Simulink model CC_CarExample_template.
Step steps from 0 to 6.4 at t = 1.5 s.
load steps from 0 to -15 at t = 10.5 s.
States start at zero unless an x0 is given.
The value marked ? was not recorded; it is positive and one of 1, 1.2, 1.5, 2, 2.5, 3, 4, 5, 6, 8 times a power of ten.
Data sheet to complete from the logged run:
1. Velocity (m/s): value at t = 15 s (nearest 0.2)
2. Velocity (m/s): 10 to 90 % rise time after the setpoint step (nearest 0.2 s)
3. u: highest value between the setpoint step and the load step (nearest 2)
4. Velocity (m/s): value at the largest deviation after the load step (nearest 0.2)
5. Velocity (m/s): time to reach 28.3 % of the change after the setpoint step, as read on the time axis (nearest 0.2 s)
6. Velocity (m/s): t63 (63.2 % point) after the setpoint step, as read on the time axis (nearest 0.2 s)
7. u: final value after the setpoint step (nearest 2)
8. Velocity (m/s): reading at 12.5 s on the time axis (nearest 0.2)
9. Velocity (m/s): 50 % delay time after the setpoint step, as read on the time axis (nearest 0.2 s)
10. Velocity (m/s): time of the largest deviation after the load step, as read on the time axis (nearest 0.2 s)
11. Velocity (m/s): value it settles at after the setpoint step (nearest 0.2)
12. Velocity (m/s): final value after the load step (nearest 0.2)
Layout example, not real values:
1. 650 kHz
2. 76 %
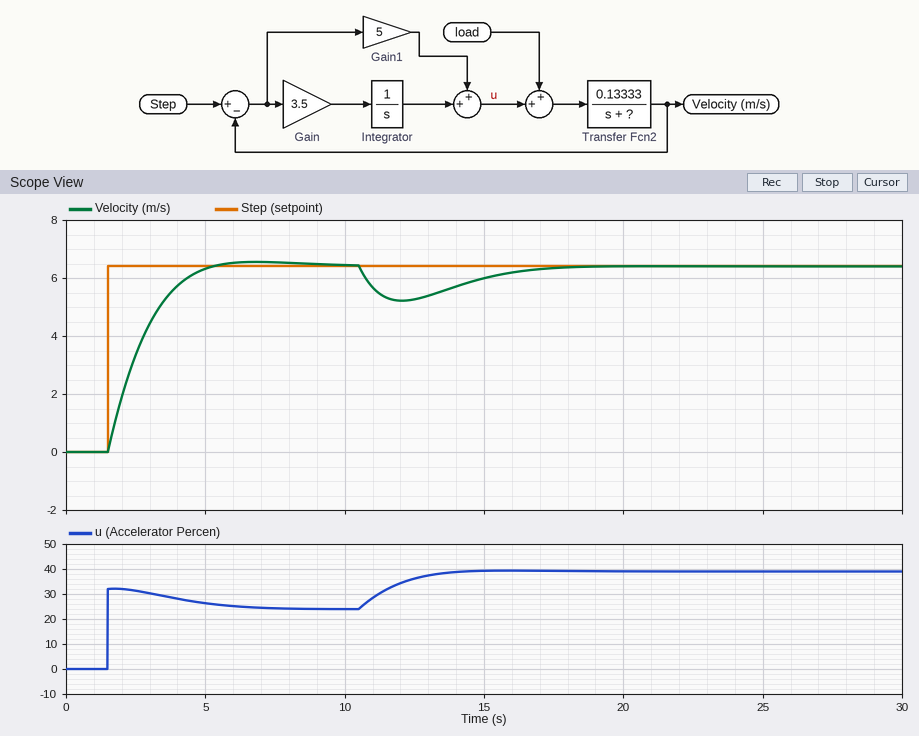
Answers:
1. 6.0
2. 2.4 s
3. 32
4. 5.2
5. 2.0 s
6. 2.8 s
7. 24
8. 5.2
9. 2.4 s
10. 12.0 s
11. 6.4
12. 6.4
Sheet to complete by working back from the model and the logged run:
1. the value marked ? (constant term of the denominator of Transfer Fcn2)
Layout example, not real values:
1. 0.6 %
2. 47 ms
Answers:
1. 0.5
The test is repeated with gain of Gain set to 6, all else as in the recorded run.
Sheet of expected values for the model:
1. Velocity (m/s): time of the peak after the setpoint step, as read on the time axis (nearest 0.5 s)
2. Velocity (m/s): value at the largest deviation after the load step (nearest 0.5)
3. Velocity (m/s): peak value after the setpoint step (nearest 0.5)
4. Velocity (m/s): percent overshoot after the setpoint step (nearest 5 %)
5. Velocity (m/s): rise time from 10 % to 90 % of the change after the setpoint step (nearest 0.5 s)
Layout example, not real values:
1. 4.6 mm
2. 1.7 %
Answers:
1. 5.0 s
2. 5.5
3. 7.0
4. 10 %
5. 1.5 s
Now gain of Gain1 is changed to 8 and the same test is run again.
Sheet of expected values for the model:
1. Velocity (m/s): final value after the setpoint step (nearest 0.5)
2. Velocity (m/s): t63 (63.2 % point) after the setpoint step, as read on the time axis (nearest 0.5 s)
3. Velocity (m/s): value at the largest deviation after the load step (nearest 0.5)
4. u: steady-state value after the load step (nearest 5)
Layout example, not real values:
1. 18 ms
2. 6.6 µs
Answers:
1. 6.5
2. 2.5 s
3. 5.5
4. 40
